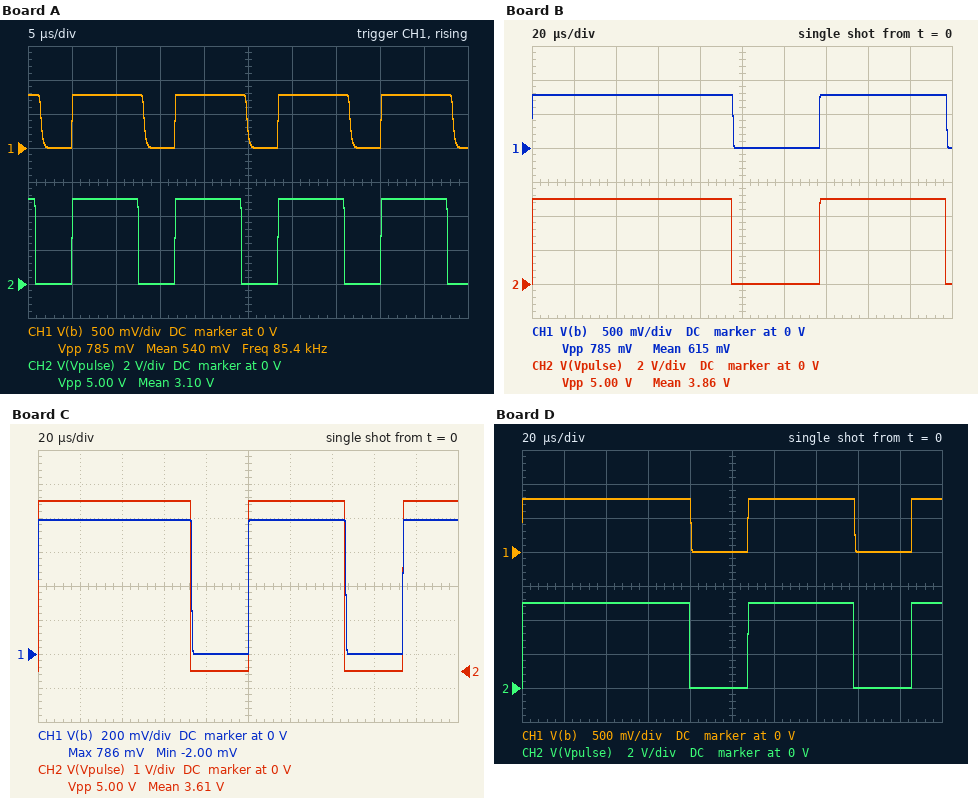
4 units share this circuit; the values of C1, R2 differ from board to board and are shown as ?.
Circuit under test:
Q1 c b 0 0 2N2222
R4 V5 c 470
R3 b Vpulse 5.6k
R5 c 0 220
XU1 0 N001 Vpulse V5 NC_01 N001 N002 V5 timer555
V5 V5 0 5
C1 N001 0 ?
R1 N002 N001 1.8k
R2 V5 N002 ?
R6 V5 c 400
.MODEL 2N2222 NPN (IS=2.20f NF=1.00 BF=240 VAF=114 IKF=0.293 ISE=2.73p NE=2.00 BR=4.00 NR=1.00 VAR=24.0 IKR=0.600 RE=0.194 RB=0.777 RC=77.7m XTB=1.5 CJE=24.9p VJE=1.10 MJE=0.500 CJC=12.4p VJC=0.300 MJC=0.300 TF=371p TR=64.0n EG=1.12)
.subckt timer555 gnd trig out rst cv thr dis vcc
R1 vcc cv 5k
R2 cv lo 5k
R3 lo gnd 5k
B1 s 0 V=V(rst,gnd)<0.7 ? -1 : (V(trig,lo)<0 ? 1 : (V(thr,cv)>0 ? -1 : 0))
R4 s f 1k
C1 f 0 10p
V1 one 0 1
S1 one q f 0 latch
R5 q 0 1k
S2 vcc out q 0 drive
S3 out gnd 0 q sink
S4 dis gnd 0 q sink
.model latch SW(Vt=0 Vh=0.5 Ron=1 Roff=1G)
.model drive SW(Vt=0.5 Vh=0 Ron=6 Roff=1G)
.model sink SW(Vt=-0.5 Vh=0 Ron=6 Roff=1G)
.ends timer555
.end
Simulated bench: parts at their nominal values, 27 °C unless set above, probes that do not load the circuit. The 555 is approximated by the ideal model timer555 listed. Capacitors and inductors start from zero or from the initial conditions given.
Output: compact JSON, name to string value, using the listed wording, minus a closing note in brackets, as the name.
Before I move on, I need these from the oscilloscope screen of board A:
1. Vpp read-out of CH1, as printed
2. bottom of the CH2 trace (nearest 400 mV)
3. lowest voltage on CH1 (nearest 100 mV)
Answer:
{"Vpp read-out of CH1, as printed": "785 mV", "bottom of the CH2 trace": "0 V", "lowest voltage on CH1": "0 V"}
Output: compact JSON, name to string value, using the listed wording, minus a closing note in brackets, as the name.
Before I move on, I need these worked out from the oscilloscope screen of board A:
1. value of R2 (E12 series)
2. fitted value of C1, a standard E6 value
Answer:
{"value of R2": "1.5 kΩ", "fitted value of C1, a standard E6 value": "3.3 nF"}
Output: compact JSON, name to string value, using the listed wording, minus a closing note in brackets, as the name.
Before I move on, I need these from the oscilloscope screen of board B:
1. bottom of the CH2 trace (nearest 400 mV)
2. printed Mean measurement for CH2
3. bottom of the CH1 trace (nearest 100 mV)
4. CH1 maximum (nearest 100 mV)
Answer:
{"bottom of the CH2 trace": "0 V", "printed Mean measurement for CH2": "3.86 V", "bottom of the CH1 trace": "0 V", "CH1 maximum": "800 mV"}
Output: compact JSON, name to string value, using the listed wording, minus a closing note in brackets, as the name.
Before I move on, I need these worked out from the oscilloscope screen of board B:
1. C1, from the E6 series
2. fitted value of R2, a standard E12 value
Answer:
{"C1, from the E6 series": "33 nF", "fitted value of R2, a standard E12 value": "820 Ω"}
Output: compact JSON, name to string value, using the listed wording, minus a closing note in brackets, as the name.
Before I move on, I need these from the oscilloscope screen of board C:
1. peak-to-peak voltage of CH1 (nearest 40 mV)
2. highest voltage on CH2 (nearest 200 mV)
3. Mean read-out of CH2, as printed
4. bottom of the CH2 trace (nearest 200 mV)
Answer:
{"peak-to-peak voltage of CH1": "800 mV", "highest voltage on CH2": "5.0 V", "Mean read-out of CH2, as printed": "3.61 V", "bottom of the CH2 trace": "0 V"}
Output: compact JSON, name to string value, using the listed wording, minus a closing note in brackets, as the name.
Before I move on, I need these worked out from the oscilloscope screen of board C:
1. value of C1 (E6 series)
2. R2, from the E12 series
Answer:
{"value of C1": "22 nF", "R2, from the E12 series": "1.2 kΩ"}
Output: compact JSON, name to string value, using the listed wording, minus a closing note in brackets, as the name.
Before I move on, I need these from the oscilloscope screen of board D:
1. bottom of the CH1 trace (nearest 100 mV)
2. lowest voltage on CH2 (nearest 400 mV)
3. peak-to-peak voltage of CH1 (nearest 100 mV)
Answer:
{"bottom of the CH1 trace": "0 V", "lowest voltage on CH2": "0 V", "peak-to-peak voltage of CH1": "800 mV"}
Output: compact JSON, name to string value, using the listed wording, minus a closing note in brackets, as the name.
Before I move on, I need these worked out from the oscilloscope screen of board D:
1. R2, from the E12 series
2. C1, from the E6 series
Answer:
{"R2, from the E12 series": "1.5 kΩ", "C1, from the E6 series": "22 nF"}
